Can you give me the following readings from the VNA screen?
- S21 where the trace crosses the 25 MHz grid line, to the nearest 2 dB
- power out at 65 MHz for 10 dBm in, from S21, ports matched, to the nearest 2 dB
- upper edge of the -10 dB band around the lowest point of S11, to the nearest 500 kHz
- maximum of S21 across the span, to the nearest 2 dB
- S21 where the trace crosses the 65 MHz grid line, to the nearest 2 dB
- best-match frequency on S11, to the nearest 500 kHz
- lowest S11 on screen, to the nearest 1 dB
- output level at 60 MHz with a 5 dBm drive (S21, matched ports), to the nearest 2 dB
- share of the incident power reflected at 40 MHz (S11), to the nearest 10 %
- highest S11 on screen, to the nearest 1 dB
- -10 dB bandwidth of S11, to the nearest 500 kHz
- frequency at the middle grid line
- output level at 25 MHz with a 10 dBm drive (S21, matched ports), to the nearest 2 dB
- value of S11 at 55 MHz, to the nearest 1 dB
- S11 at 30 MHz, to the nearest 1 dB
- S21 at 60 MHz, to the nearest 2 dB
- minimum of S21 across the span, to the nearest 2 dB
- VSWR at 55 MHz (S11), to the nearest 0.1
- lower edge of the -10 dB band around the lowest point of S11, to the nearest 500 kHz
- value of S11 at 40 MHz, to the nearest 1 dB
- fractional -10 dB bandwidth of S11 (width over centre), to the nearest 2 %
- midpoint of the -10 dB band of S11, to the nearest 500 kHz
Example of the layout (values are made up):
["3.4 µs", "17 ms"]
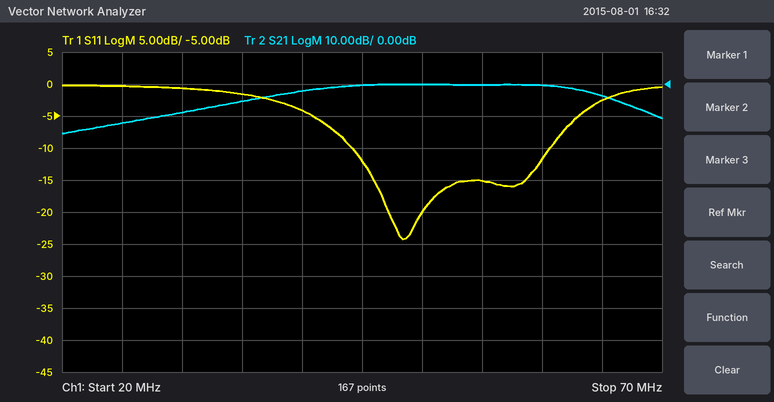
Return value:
["-12 dB", "6 dBm", "60.5 MHz", "0 dB", "-4 dB", "48.5 MHz", "-24 dB", "4 dBm", "40 %", "0 dB", "16.5 MHz", "45 MHz", "-2 dBm", "-15 dB", "-1 dB", "0 dB", "-16 dB", "1.4", "44.0 MHz", "-4 dB", "32 %", "52.5 MHz"]
